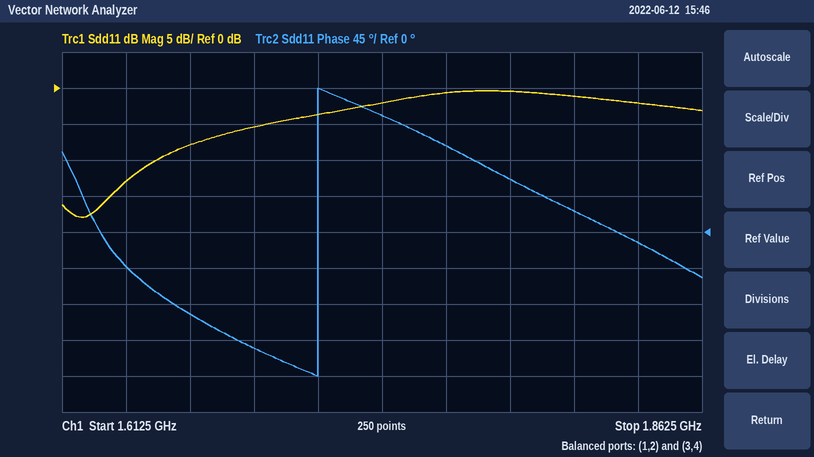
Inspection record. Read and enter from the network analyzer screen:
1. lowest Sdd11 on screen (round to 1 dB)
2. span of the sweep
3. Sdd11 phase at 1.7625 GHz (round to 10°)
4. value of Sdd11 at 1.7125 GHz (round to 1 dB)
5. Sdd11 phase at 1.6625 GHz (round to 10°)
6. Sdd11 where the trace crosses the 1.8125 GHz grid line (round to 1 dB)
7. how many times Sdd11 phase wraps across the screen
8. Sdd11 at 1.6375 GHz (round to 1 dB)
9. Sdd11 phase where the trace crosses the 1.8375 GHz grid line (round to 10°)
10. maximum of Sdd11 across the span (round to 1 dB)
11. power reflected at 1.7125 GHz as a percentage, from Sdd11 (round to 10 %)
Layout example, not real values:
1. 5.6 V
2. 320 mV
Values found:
1. -18 dB
2. 250 MHz
3. 110°
4. -4 dB
5. -100°
6. -1 dB
7. 1
8. -13 dB
9. -10°
10. 0 dB
11. 40 %
